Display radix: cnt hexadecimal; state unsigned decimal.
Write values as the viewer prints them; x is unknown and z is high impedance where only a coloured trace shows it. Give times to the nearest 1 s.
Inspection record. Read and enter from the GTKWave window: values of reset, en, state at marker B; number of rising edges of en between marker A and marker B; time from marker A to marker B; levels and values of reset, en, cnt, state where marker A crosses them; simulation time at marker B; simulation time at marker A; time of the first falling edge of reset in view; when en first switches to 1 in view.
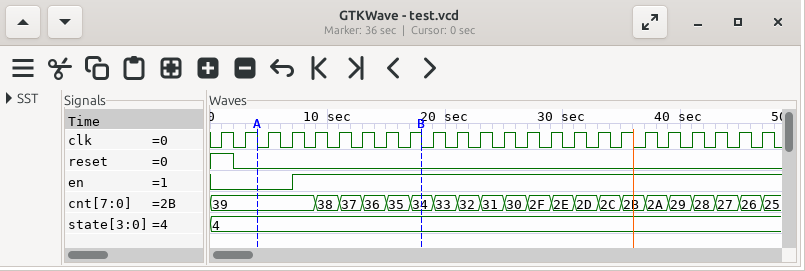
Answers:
reset=0, en=1, state=4
1
14 s
reset=0, en=0, cnt=39, state=4
18 s
4 s
2 s
7 s
